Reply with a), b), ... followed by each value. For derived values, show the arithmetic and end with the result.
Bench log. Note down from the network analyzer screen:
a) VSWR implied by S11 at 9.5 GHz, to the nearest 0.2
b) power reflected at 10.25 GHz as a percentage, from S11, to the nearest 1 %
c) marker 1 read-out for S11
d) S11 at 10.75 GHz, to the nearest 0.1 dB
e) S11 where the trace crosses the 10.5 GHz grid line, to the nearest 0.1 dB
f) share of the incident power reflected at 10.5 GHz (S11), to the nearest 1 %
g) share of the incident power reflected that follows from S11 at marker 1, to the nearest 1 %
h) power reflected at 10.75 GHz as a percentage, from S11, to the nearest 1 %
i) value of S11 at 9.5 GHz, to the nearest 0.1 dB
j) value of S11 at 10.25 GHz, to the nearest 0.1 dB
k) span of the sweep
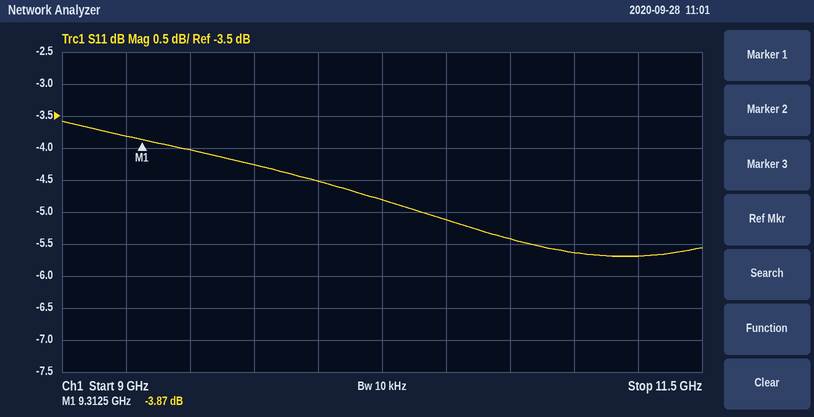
a) |Γ| = 10^(-4/20) = 0.6310; VSWR = (1 + 0.6310)/(1 − 0.6310) ≈ 4.4
b) 10^(-4.8/10) ≈ 33 %
c) -3.87 dB
d) -5.4 dB
e) -5.1 dB
f) 10^(-5.1/10) ≈ 31 %
g) 10^(-3.87/10) ≈ 41 %
h) 10^(-5.4/10) ≈ 29 %
i) -4.0 dB
j) -4.8 dB
k) 2.5 GHz
